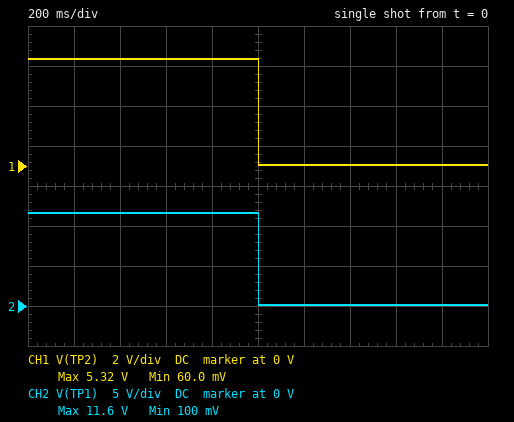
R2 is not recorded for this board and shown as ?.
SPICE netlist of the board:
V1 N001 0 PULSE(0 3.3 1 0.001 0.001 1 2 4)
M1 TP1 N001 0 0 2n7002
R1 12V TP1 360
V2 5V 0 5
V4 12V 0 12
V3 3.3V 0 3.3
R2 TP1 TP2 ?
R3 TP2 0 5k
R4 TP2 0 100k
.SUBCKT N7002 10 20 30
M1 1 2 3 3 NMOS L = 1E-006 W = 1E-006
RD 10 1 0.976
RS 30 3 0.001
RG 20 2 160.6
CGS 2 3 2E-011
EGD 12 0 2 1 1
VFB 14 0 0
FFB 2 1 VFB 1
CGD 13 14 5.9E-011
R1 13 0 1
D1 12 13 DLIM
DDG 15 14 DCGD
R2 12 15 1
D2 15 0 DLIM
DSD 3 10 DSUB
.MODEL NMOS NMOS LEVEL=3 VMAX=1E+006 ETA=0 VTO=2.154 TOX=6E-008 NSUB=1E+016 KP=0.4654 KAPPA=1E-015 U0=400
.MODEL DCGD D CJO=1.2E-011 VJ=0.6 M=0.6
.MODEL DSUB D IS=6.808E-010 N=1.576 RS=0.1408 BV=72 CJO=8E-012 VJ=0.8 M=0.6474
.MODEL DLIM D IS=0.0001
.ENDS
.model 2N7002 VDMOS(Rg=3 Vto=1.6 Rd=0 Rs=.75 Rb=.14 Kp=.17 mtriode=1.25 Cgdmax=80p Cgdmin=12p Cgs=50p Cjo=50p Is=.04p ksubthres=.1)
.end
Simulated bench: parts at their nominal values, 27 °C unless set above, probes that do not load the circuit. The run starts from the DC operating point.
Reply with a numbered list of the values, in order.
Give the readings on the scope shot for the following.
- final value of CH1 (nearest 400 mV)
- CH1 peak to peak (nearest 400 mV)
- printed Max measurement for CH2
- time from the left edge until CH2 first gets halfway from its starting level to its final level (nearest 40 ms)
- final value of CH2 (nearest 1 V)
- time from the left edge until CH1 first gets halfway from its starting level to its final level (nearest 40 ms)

1. 0 V
2. 5.2 V
3. 11.6 V
4. 1.00 s
5. 0 V
6. 1.00 s
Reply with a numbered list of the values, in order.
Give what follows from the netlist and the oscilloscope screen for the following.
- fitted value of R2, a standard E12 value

1. 5.6 kΩ
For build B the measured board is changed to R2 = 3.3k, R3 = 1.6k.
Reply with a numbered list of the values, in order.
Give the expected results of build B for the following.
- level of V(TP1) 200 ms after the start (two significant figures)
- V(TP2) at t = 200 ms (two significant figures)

1. 11 V
2. 3.6 V
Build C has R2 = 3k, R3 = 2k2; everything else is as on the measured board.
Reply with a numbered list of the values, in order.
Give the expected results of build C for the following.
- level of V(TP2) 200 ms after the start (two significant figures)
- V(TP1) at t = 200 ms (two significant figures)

1. 4.7 V
2. 11 V
